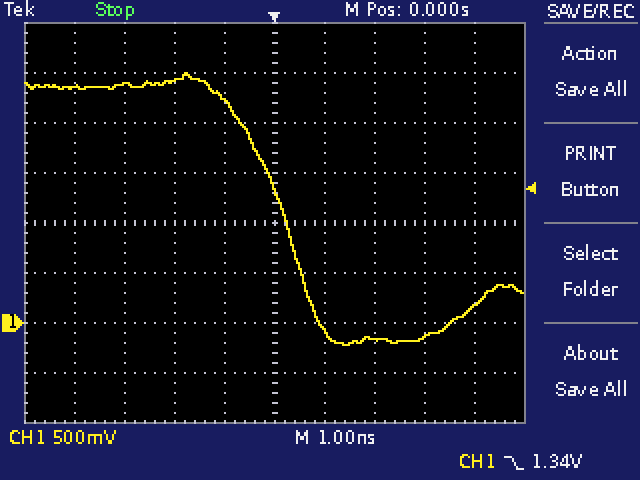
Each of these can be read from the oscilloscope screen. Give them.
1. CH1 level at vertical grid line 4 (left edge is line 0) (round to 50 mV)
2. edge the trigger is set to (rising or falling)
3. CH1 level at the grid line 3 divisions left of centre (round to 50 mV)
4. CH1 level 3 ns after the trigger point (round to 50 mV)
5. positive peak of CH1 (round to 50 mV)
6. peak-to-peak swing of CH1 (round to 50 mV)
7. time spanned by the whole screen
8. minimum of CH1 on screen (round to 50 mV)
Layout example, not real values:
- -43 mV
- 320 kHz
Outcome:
- 2.25 V
- falling
- 2.40 V
- -150 mV
- 2.50 V
- 2.70 V
- 10 ns
- -200 mV
